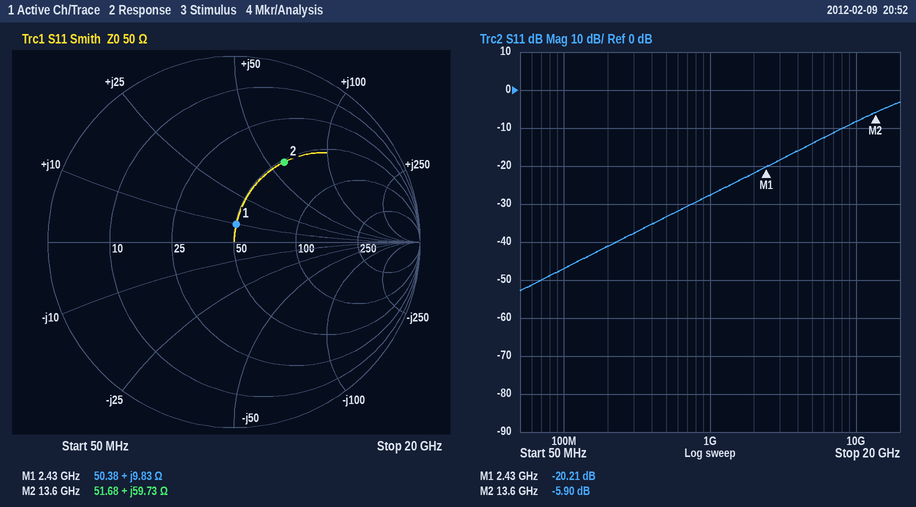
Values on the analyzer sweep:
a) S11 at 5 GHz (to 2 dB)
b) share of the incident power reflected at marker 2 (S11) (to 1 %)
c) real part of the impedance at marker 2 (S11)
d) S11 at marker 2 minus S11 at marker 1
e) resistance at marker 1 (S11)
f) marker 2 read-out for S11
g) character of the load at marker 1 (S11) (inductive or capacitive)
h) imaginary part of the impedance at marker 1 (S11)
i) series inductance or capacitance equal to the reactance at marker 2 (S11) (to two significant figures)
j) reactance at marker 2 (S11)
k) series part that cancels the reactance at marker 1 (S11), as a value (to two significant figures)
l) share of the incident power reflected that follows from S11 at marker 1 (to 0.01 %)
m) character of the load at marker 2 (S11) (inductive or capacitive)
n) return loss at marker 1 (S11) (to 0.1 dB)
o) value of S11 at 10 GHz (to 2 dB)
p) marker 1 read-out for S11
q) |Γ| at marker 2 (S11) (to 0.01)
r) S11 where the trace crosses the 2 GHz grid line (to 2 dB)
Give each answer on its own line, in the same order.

-14 dB
26 %
51.68 Ω
14.31 dB
50.38 Ω
-5.90 dB
inductive
+9.83 Ω
700 pH
+59.73 Ω
6.7 pF
0.95 %
inductive
20.2 dB
-8 dB
-20.21 dB
0.51
-22 dB
